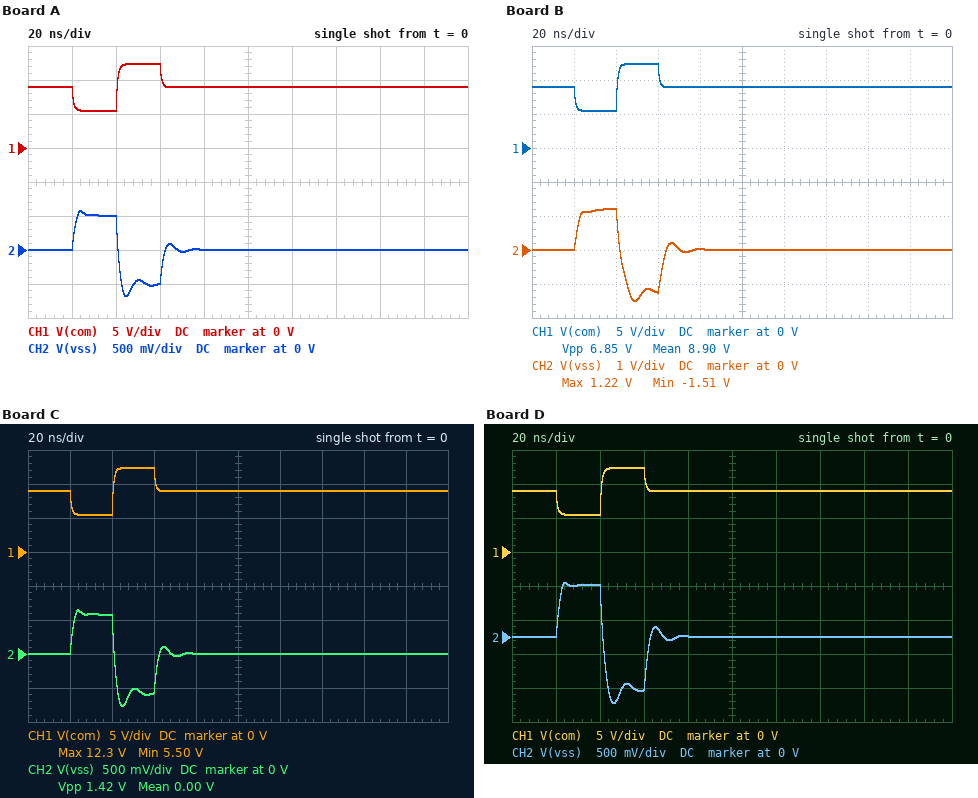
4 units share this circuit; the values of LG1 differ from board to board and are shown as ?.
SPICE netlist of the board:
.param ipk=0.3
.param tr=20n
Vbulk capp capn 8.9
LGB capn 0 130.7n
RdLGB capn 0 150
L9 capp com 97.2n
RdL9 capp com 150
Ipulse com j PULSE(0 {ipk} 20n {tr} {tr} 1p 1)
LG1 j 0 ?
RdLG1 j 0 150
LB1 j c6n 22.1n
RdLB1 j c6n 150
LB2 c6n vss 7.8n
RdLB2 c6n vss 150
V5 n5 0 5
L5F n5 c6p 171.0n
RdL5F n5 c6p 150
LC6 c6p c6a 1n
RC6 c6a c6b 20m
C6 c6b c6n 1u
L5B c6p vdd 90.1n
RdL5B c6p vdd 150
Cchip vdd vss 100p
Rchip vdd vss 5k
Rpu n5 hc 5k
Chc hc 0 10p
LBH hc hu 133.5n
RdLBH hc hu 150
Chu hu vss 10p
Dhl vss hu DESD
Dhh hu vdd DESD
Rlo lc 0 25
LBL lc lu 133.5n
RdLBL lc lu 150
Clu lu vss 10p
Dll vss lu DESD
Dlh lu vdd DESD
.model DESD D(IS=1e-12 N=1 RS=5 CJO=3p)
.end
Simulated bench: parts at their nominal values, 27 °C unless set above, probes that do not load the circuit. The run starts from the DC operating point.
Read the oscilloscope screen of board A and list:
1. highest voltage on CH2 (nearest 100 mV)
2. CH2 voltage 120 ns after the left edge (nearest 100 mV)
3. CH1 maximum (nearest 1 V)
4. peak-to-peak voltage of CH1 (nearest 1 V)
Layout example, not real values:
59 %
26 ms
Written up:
600 mV
0 V
12 V
7 V
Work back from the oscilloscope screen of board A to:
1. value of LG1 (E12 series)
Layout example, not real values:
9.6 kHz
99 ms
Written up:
47 nH
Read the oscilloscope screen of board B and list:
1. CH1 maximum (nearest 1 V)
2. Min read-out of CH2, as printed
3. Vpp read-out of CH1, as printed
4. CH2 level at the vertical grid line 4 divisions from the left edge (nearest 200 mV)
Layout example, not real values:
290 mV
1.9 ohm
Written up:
12 V
-1.51 V
6.85 V
0 V
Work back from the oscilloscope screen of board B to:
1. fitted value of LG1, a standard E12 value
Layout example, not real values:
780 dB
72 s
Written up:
180 nH
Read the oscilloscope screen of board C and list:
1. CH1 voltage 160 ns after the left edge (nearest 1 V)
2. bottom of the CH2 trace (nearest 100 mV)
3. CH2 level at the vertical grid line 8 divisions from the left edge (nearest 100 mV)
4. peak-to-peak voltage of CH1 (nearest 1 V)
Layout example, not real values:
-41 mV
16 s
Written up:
9 V
-800 mV
0 V
7 V
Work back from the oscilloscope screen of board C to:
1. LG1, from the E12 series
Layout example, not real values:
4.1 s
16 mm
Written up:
56 nH
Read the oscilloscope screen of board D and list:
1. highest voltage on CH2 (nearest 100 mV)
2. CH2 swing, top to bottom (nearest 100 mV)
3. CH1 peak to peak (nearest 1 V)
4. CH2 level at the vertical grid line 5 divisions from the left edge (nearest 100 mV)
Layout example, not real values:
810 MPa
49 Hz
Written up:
800 mV
1.8 V
7 V
0 V
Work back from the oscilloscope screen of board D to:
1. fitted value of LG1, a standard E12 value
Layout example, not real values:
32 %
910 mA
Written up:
82 nH
